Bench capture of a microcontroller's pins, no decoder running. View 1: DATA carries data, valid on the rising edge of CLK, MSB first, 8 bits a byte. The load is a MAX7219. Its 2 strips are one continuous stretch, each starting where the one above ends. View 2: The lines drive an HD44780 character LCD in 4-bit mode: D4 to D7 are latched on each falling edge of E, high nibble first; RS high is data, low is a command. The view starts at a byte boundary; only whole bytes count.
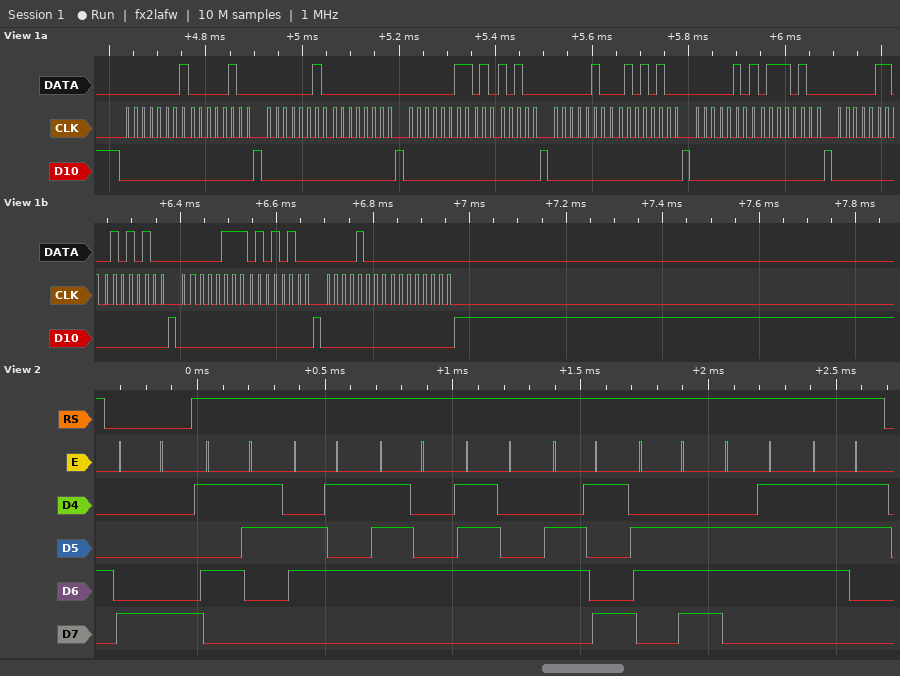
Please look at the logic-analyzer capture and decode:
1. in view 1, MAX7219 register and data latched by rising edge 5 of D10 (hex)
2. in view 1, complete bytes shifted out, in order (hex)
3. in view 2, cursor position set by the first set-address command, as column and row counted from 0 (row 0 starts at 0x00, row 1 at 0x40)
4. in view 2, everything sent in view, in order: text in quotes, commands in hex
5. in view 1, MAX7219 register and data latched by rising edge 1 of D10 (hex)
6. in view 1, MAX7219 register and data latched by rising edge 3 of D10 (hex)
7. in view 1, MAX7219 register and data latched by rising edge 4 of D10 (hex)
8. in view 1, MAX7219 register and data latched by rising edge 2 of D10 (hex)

register 0x5, data 0x74
01 04 02 00 03 54 04 54 05 74 06 54 07 54 08 00
column 8, row 0
0x88 "Settings"
register 0x1, data 0x04
register 0x3, data 0x54
register 0x4, data 0x54
register 0x2, data 0x00
